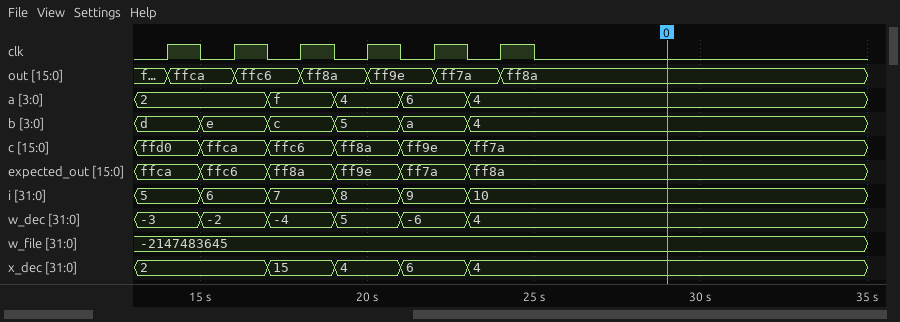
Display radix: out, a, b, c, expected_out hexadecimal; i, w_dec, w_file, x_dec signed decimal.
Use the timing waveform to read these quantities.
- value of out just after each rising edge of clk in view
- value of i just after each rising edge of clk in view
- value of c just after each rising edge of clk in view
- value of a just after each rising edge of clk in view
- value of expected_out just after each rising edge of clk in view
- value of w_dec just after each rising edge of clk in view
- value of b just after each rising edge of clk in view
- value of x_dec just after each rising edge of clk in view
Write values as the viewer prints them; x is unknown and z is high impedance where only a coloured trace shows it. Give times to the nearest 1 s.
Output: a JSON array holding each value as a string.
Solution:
["ffca, ffc6, ff8a, ff9e, ff7a, ff8a", "5, 6, 7, 8, 9, 10", "ffd0, ffca, ffc6, ff8a, ff9e, ff7a", "2, 2, f, 4, 6, 4", "ffca, ffc6, ff8a, ff9e, ff7a, ff8a", "-3, -2, -4, 5, -6, 4", "d, e, c, 5, a, 4", "2, 2, 15, 4, 6, 4"]
